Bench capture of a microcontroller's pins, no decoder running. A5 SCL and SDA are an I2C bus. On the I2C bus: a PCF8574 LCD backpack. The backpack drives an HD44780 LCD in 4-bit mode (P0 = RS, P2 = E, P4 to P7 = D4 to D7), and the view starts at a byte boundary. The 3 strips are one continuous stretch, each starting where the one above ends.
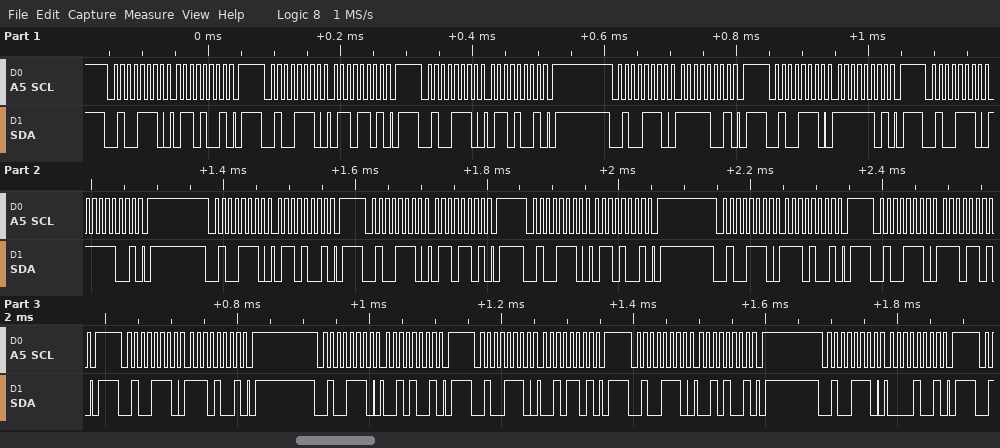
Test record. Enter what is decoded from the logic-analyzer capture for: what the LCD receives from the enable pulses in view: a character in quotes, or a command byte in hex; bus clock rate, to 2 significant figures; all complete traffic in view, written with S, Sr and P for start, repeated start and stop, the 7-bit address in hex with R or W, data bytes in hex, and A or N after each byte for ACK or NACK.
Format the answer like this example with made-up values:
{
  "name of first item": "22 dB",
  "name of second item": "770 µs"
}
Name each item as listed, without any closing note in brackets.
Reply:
{
  "what the LCD receives from the enable pulses in view: a character in quotes, or a command byte in hex": "'o' 'n'",
  "bus clock rate, to 2 significant figures": "100 kHz",
  "all complete traffic in view, written with S, Sr and P for start, repeated start and stop, the 7-bit address in hex with R or W, data bytes in hex, and A or N after each byte for ACK or NACK": "S 27W A 69 A P S 27W A 6D A P S 27W A 69 A P S 27W A F9 A P S 27W A FD A P S 27W A F9 A P S 27W A 69 A P S 27W A 6D A P S 27W A 69 A P S 27W A E9 A P S 27W A ED A P S 27W A E9 A P S 27W A 29 A P S 27W A 2D A P S 27W A 29 A P S 27W A 09 A P"
}
